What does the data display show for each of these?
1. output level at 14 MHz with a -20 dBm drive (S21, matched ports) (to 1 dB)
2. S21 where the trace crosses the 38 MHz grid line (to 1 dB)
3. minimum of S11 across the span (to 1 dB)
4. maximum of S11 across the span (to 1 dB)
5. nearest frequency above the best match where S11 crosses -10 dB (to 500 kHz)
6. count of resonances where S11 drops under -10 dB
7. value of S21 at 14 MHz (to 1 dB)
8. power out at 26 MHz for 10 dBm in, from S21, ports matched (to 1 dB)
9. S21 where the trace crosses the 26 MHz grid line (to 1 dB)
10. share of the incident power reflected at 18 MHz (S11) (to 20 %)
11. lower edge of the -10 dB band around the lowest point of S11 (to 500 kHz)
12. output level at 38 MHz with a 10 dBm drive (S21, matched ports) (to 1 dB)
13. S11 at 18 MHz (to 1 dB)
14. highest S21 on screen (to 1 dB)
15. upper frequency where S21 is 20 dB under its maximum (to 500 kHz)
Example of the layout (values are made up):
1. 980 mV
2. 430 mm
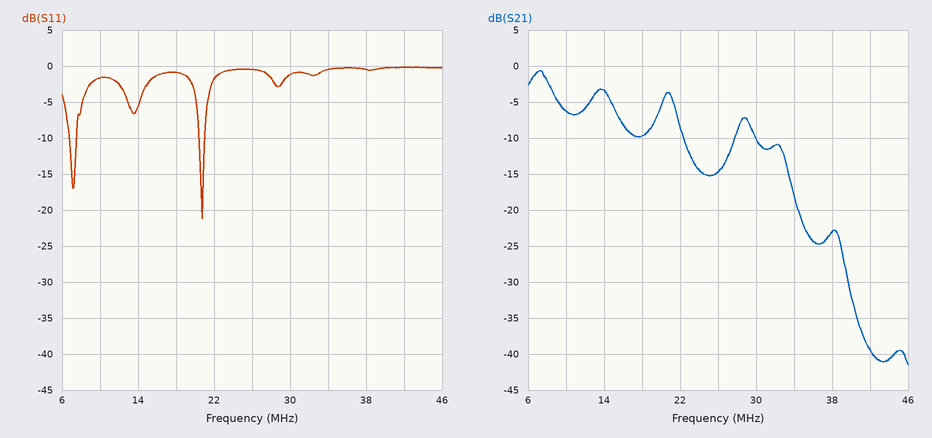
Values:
1. -23 dBm
2. -23 dB
3. -21 dB
4. 0 dB
5. 21.0 MHz
6. 2
7. -3 dB
8. -5 dBm
9. -15 dB
10. 80 %
11. 20.5 MHz
12. -13 dBm
13. -1 dB
14. -1 dB
15. 34.5 MHz
